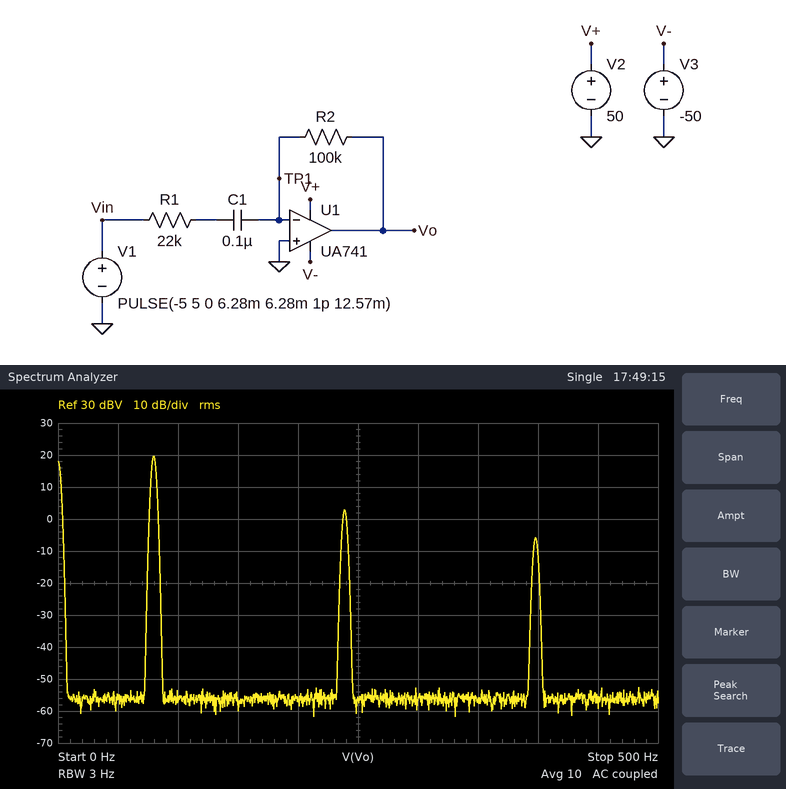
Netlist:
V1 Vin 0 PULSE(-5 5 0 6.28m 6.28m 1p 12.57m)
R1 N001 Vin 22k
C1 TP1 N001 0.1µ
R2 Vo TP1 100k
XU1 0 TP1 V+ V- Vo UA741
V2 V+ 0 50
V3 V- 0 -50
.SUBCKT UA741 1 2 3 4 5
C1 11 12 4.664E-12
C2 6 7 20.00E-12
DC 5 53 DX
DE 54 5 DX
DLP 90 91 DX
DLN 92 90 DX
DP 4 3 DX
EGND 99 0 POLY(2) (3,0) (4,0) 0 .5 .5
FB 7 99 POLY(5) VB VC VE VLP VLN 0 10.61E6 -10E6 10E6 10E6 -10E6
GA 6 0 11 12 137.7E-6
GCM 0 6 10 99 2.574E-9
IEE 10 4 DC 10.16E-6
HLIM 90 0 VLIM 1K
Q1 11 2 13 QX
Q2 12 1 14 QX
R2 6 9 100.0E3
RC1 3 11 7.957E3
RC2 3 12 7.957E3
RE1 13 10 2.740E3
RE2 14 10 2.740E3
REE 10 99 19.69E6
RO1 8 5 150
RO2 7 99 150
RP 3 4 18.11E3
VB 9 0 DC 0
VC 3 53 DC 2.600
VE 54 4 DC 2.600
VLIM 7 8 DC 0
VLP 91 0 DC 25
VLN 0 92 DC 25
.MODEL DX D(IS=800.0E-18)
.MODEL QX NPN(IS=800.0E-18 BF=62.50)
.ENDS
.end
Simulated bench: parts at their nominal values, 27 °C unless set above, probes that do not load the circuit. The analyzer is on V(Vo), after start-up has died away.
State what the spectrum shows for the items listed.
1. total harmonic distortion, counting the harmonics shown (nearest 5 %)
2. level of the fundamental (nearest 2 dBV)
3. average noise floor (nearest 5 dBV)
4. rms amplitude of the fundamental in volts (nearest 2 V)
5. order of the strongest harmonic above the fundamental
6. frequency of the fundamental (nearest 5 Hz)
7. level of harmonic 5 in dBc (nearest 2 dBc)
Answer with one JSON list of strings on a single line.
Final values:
["15 %", "20 dBV", "-55 dBV", "10 V", "3", "80 Hz", "-26 dBc"]
